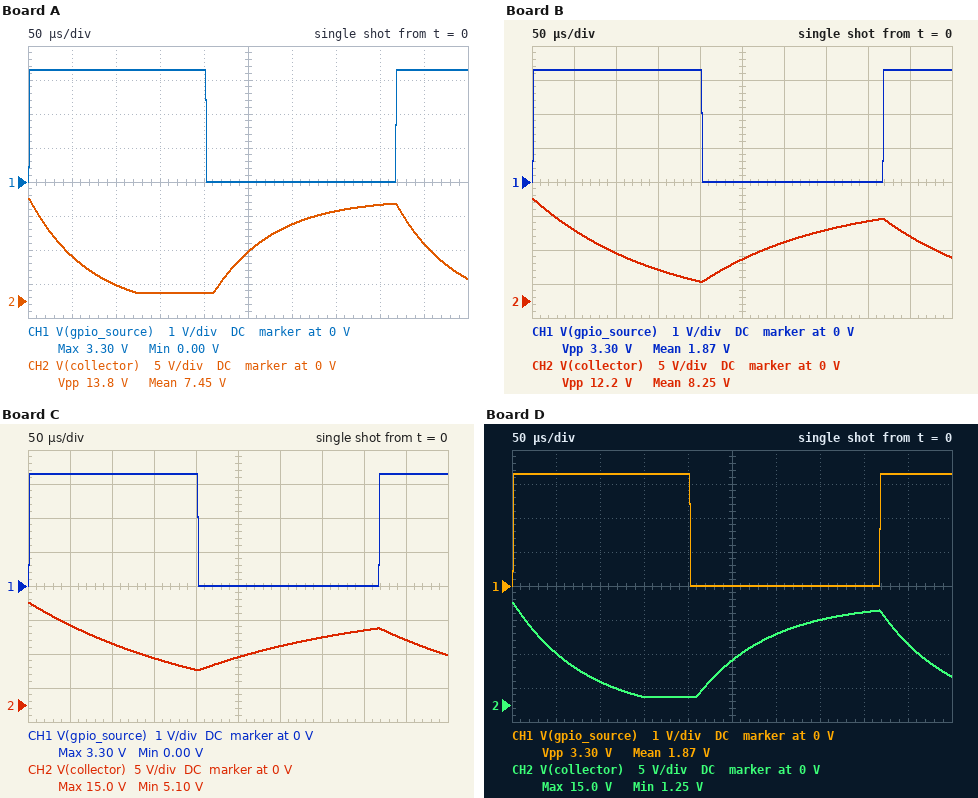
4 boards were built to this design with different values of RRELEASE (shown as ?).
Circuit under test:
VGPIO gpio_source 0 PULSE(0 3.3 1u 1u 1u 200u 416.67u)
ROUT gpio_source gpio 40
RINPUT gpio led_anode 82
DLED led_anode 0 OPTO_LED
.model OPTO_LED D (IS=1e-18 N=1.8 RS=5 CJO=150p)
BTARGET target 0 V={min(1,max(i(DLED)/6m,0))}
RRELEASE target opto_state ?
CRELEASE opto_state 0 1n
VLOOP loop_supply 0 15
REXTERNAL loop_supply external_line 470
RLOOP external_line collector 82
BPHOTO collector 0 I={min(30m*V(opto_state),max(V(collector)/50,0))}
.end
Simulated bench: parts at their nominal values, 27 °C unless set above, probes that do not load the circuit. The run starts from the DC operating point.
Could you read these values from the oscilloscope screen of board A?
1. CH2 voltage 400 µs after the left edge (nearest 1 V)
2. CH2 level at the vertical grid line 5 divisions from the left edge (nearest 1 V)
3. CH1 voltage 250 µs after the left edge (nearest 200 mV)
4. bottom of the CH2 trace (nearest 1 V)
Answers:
14 V
7 V
0 V
1 V
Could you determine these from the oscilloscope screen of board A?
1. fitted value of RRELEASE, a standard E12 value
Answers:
68 kΩ
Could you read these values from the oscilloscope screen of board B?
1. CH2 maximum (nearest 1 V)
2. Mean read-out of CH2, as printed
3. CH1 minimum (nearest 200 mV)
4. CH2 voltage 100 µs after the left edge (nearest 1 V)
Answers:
15 V
8.25 V
0 V
7 V
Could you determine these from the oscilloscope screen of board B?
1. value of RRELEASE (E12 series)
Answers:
150 kΩ
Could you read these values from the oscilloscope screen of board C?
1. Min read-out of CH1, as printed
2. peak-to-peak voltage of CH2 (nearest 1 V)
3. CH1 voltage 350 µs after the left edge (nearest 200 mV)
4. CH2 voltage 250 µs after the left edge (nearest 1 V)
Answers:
0.00 V
10 V
0 V
7 V
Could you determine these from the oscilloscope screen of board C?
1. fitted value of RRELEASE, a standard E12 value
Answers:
220 kΩ
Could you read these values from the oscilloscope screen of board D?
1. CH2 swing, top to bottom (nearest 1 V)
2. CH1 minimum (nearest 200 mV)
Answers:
14 V
0 V
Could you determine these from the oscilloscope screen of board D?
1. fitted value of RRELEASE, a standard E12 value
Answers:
82 kΩ
